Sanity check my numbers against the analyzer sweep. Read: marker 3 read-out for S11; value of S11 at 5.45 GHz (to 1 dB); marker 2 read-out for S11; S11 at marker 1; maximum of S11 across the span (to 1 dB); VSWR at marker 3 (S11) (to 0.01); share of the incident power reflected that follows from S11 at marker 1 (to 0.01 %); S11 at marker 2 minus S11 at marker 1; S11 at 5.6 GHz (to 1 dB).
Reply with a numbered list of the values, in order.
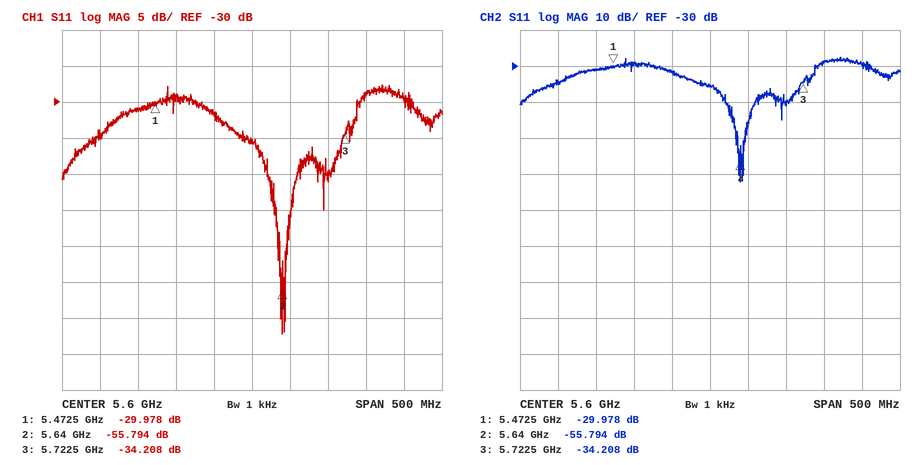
1. -34.208 dB
2. -31 dB
3. -55.794 dB
4. -29.978 dB
5. -28 dB
6. 1.04
7. 0.10 %
8. -25.816 dB
9. -35 dB
